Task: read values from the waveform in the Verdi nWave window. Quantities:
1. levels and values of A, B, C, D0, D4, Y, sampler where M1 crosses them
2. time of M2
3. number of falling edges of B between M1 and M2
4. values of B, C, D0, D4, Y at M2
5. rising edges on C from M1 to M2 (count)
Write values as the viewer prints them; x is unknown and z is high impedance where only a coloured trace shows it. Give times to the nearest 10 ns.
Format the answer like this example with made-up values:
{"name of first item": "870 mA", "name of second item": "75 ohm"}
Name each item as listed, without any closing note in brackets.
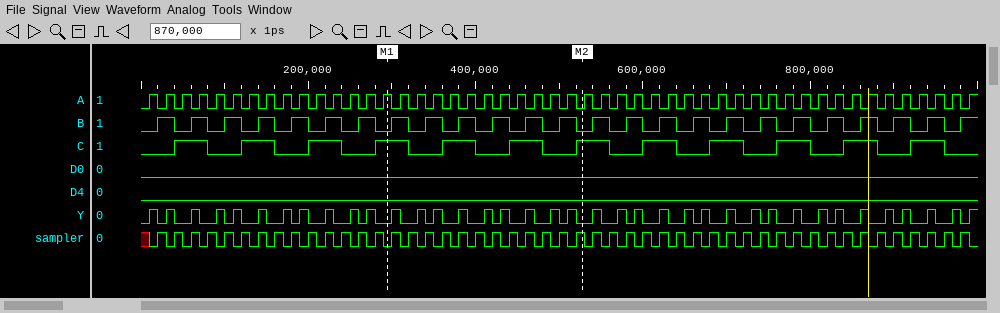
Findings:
{"levels and values of A, B, C, D0, D4, Y, sampler where M1 crosses them": "A=1, B=0, C=1, D0=0, D4=0, Y=0, sampler=0", "time of M2": "530 ns", "number of falling edges of B between M1 and M2": "6", "values of B, C, D0, D4, Y at M2": "B=0, C=1, D0=0, D4=0, Y=0", "rising edges on C from M1 to M2": "3"}
